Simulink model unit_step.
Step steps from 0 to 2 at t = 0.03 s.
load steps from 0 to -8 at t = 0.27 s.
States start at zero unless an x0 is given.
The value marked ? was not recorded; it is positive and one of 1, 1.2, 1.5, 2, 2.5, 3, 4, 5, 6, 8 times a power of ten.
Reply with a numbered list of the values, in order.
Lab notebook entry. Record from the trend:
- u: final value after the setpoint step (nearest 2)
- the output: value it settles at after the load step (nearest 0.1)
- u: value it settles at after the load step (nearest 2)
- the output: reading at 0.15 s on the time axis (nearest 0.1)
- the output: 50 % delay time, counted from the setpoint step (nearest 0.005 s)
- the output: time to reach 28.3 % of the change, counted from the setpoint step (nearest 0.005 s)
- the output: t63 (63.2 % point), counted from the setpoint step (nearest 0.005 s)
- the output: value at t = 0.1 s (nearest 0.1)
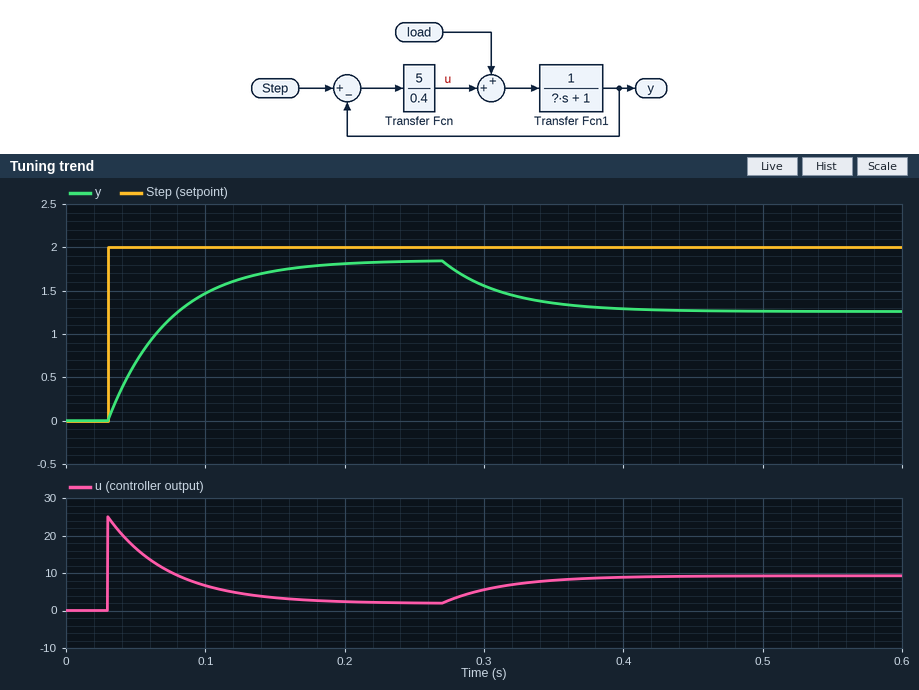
1. 2
2. 1.3
3. 10
4. 1.7
5. 0.030 s
6. 0.015 s
7. 0.045 s
8. 1.5
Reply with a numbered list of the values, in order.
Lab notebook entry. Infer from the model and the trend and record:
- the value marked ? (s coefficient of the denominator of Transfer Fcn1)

1. 0.6
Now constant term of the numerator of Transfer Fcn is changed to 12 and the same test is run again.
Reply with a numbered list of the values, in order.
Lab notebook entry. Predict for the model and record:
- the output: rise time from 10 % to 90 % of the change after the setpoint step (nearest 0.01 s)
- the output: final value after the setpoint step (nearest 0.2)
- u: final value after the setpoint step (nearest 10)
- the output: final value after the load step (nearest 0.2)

1. 0.04 s
2. 2.0
3. 0
4. 1.6
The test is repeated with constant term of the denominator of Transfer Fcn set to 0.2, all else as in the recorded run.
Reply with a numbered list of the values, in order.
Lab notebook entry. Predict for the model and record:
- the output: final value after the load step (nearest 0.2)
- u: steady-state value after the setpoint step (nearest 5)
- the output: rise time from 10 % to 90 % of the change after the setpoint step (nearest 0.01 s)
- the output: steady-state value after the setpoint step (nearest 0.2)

1. 1.6
2. 0
3. 0.05 s
4. 2.0
